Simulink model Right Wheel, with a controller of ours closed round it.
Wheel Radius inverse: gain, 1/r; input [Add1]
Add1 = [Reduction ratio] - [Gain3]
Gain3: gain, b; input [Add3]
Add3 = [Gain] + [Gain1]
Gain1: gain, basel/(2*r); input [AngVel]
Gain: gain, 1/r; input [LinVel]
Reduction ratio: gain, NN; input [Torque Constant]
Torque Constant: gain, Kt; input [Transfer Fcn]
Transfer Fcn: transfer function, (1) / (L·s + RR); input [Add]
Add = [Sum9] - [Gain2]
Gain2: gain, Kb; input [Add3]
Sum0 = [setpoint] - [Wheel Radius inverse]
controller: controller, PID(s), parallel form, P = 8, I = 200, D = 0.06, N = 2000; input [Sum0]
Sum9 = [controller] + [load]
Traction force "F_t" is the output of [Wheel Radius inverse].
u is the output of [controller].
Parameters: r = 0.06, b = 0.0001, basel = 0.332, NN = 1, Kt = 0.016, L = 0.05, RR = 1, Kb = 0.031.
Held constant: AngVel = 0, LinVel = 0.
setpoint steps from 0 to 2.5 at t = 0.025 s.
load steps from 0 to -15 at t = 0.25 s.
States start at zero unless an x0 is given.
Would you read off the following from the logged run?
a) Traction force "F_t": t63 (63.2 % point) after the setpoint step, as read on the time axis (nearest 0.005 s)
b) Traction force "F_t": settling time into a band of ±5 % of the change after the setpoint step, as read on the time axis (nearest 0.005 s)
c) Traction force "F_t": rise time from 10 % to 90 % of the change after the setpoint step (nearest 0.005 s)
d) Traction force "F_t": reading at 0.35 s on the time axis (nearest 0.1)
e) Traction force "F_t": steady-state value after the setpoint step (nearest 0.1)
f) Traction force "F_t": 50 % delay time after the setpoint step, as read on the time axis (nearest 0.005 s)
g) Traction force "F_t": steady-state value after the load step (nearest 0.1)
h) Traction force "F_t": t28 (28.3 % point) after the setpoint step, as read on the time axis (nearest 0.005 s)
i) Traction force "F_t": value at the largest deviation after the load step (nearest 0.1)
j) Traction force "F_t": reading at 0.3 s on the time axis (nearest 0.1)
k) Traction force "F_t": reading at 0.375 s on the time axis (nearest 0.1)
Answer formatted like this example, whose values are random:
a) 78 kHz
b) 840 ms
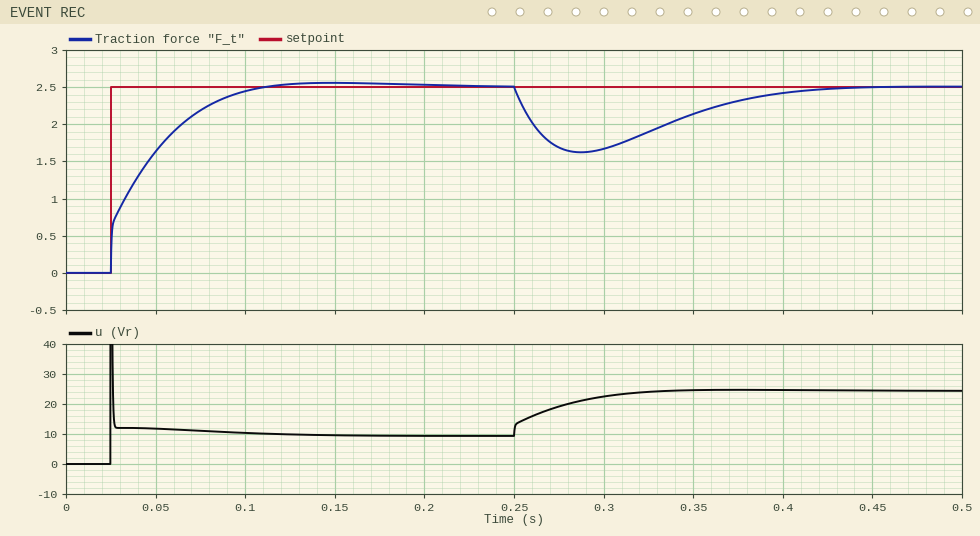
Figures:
a) 0.050 s
b) 0.090 s
c) 0.055 s
d) 2.1
e) 2.5
f) 0.040 s
g) 2.5
h) 0.025 s
i) 1.6
j) 1.7
k) 2.3
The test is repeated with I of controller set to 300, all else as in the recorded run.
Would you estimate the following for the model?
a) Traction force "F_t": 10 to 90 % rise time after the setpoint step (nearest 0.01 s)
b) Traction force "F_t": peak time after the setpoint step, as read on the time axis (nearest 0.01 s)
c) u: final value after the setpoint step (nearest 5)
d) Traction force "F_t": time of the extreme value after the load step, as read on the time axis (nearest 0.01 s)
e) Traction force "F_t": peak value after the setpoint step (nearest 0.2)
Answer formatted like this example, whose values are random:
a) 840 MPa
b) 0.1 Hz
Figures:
a) 0.04 s
b) 0.11 s
c) 10
d) 0.28 s
e) 2.6
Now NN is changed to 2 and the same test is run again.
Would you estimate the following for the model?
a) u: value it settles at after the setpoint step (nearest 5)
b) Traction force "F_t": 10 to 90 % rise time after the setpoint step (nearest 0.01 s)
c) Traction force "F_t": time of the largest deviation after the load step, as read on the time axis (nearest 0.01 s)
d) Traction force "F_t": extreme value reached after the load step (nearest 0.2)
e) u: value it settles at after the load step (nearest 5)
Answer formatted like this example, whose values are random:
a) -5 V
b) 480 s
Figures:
a) 5
b) 0.03 s
c) 0.28 s
d) 1.4
e) 20
